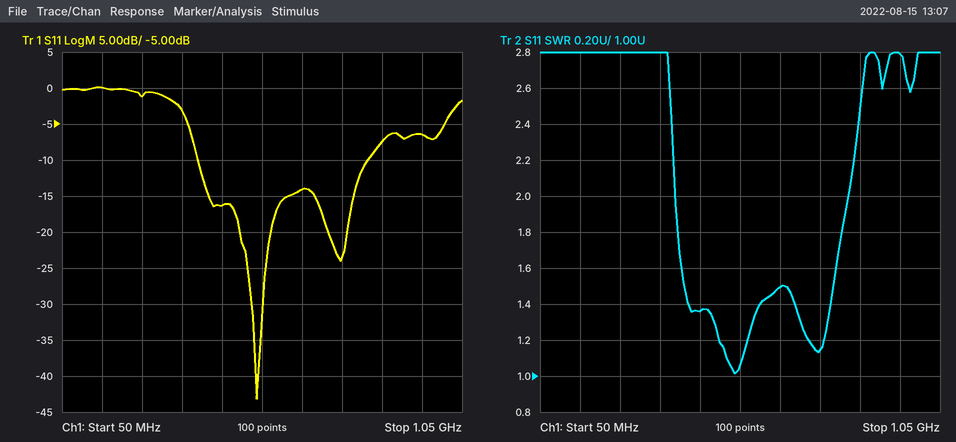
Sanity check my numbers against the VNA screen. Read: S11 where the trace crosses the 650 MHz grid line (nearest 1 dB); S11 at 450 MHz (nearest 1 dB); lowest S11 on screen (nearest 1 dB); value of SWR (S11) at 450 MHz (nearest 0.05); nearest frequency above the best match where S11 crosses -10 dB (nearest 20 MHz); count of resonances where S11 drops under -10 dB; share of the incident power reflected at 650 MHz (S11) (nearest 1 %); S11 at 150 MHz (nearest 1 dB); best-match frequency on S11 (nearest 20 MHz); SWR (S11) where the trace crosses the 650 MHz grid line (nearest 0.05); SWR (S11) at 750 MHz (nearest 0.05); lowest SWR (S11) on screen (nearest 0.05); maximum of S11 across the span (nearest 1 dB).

-14 dB
-16 dB
-43 dB
1.35
820 MHz
2
4 %
0 dB
540 MHz
1.50
1.15
1.00
0 dB
